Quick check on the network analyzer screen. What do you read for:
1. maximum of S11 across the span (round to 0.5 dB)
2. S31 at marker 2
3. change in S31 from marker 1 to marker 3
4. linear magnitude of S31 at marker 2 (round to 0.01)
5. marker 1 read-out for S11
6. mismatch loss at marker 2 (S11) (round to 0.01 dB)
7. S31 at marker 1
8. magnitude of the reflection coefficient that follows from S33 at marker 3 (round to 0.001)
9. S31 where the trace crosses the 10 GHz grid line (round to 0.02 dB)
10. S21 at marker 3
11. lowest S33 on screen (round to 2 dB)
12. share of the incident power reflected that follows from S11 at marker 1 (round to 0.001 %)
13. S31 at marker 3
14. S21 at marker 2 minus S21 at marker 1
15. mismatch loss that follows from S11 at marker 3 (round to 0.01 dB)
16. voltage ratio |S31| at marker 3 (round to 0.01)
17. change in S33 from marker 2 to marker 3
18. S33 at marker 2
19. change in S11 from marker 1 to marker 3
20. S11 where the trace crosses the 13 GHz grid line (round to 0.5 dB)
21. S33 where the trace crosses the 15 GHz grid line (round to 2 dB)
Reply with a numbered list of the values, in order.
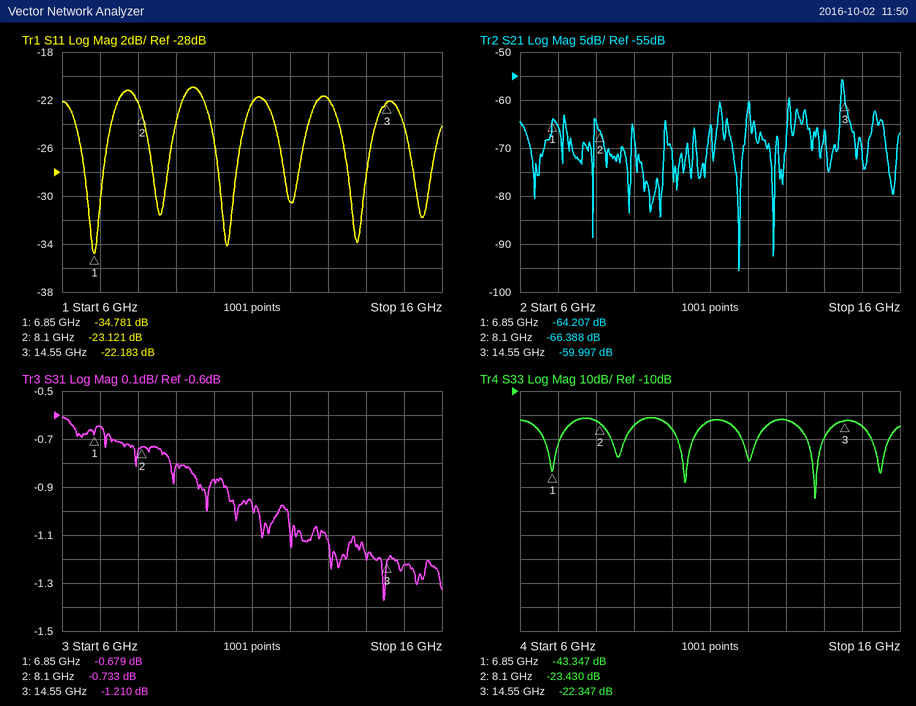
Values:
1. -21.0 dB
2. -0.733 dB
3. -0.531 dB
4. 0.92
5. -34.781 dB
6. 0.02 dB
7. -0.679 dB
8. 0.076
9. -0.88 dB
10. -59.997 dB
11. -54 dB
12. 0.033 %
13. -1.210 dB
14. -2.181 dB
15. 0.03 dB
16. 0.87
17. 1.083 dB
18. -23.430 dB
19. 12.598 dB
20. -22.0 dB
21. -24 dB
